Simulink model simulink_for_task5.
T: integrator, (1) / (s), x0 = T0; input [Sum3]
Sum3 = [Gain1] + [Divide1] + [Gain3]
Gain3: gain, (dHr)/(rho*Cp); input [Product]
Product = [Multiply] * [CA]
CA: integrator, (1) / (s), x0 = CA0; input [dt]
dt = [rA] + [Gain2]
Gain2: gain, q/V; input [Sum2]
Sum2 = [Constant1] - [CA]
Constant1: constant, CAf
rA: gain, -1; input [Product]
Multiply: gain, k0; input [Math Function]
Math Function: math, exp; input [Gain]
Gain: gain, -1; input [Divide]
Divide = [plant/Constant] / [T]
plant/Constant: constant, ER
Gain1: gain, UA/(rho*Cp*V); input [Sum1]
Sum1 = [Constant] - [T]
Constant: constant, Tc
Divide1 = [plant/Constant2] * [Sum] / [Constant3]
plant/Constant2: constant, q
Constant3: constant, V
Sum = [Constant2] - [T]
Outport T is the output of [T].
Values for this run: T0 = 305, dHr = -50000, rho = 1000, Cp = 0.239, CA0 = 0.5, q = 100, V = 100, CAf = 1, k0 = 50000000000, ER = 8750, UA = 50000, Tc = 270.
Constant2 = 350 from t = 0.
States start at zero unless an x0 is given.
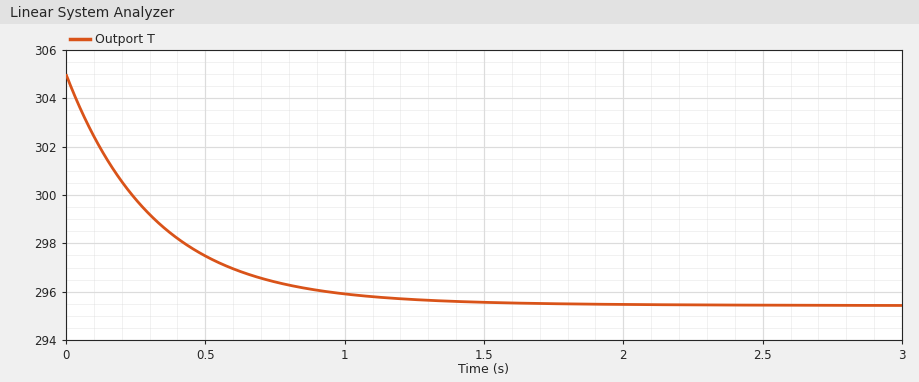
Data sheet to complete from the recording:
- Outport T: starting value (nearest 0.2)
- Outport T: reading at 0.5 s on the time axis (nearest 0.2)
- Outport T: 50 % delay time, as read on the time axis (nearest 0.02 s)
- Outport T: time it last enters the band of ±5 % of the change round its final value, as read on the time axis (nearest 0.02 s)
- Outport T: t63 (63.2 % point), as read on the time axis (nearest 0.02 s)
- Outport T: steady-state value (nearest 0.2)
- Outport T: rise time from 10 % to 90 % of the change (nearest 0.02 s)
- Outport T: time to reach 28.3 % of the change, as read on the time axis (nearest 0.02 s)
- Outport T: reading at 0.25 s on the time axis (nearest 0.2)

305.0
297.4
0.22 s
1.02 s
0.32 s
295.4
0.72 s
0.10 s
299.8
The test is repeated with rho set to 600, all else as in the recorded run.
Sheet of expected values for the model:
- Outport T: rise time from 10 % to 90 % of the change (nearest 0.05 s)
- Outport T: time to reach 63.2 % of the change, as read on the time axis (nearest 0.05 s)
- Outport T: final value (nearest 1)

0.50 s
0.20 s
288
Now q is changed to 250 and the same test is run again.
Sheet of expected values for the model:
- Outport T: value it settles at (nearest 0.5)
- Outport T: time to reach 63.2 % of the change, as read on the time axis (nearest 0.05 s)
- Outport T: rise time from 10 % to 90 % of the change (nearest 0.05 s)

312.0
0.20 s
0.35 s
